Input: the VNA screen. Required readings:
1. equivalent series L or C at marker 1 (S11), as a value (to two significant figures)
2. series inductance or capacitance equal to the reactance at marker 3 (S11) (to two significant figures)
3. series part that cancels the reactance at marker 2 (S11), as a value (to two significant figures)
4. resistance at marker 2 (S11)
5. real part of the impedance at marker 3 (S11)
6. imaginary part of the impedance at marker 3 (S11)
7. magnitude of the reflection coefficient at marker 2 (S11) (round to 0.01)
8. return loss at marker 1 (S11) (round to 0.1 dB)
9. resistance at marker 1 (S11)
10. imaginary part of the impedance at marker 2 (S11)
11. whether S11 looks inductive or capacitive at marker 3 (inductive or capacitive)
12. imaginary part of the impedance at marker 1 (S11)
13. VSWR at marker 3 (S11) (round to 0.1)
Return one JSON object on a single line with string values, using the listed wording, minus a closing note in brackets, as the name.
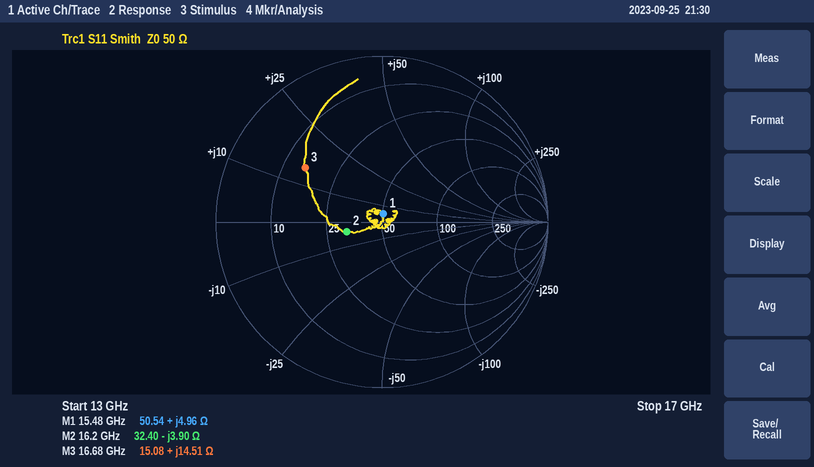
{"equivalent series L or C at marker 1 (S11), as a value": "51 pH", "series inductance or capacitance equal to the reactance at marker 3 (S11)": "140 pH", "series part that cancels the reactance at marker 2 (S11), as a value": "38 pH", "resistance at marker 2": "32.40 Ω", "real part of the impedance at marker 3": "15.08 Ω", "imaginary part of the impedance at marker 3": "+14.51 Ω", "magnitude of the reflection coefficient at marker 2 (S11)": "0.22", "return loss at marker 1 (S11)": "26.1 dB", "resistance at marker 1": "50.54 Ω", "imaginary part of the impedance at marker 2": "-3.90 Ω", "whether S11 looks inductive or capacitive at marker 3": "inductive", "imaginary part of the impedance at marker 1": "+4.96 Ω", "VSWR at marker 3 (S11)": "3.6"}
